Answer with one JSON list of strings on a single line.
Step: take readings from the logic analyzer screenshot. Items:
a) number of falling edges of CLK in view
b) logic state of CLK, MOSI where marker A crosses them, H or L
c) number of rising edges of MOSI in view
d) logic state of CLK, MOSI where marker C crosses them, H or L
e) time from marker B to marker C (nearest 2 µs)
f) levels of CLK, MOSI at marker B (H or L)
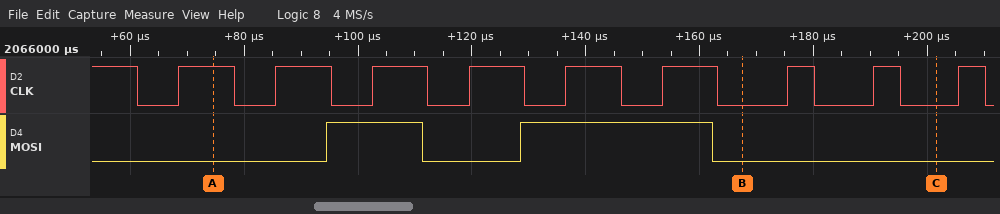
["10", "CLK=H, MOSI=L", "2", "CLK=L, MOSI=L", "34 µs", "CLK=L, MOSI=L"]
